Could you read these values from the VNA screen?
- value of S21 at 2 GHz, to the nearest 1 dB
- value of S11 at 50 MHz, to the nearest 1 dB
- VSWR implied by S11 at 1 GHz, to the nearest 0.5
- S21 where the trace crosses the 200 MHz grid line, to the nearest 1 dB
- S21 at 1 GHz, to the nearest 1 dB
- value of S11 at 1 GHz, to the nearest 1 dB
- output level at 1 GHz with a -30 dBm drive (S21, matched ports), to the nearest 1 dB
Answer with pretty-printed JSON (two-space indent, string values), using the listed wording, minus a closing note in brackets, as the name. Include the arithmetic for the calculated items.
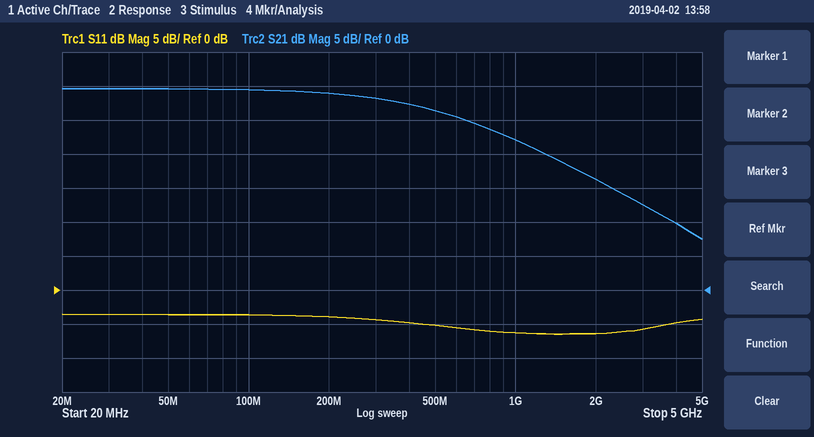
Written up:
{
  "value of S21 at 2 GHz, to the nearest 1 dB": "16 dB",
  "value of S11 at 50 MHz, to the nearest 1 dB": "-4 dB",
  "VSWR implied by S11 at 1 GHz, to the nearest 0.5": "|Γ| = 10^(-6/20) = 0.5012; VSWR = (1 + 0.5012)/(1 − 0.5012) ≈ 3.0",
  "S21 where the trace crosses the 200 MHz grid line, to the nearest 1 dB": "29 dB",
  "S21 at 1 GHz, to the nearest 1 dB": "22 dB",
  "value of S11 at 1 GHz, to the nearest 1 dB": "-6 dB",
  "output level at 1 GHz with a -30 dBm drive (S21, matched ports), to the nearest 1 dB": "-30 dBm + (22 dB) = -8 dBm"
}
